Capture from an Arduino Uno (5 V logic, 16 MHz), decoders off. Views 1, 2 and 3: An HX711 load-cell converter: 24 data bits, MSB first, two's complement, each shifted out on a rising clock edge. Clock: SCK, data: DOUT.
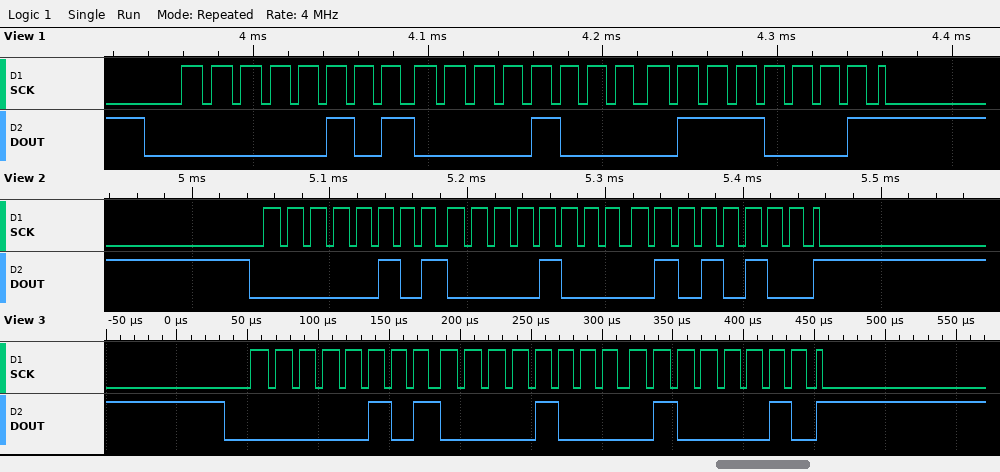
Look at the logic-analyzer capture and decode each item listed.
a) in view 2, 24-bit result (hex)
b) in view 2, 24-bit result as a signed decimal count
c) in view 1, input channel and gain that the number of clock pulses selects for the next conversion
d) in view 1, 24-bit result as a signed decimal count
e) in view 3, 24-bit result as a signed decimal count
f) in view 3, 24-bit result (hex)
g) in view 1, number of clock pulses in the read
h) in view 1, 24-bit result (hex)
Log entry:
0x050854
329812
channel A, gain 128
329841
329794
0x050842
25
0x050871
